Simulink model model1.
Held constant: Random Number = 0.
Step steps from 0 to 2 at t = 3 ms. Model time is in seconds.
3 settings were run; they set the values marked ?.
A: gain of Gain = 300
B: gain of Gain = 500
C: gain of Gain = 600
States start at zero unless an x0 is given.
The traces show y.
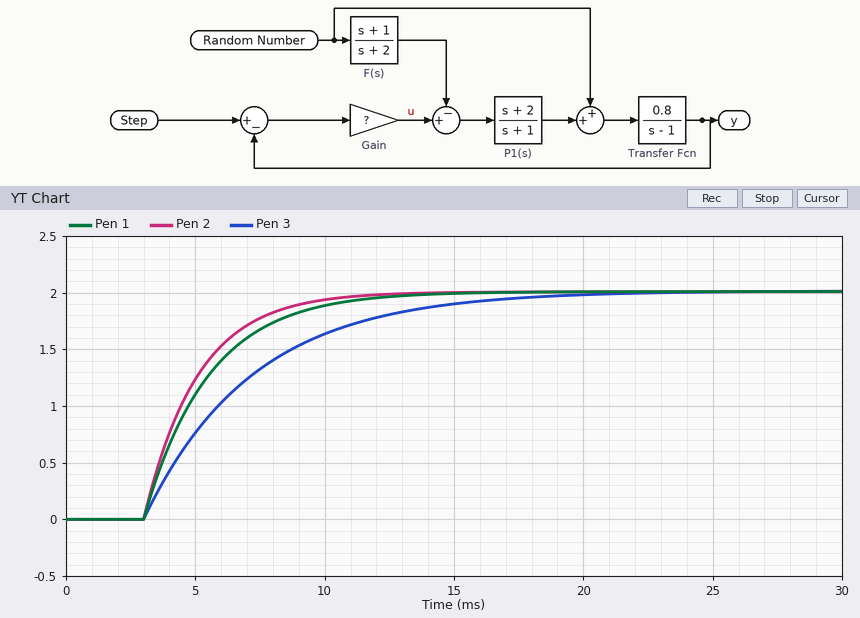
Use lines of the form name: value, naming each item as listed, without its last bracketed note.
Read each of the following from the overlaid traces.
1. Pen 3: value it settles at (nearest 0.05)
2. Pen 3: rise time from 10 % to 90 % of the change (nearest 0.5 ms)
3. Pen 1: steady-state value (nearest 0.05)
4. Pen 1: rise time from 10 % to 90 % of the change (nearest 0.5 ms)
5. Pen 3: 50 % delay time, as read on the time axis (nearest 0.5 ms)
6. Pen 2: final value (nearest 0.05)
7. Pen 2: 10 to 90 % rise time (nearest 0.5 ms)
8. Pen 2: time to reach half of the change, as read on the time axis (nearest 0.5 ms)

Pen 3: value it settles at: 2.00
Pen 3: rise time from 10 % to 90 % of the change: 9.0 ms
Pen 1: steady-state value: 2.00
Pen 1: rise time from 10 % to 90 % of the change: 5.5 ms
Pen 3: 50 % delay time, as read on the time axis: 6.0 ms
Pen 2: final value: 2.00
Pen 2: 10 to 90 % rise time: 4.5 ms
Pen 2: time to reach half of the change, as read on the time axis: 4.5 ms
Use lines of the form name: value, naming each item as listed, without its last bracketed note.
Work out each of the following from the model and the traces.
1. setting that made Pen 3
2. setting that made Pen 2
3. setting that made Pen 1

setting that made Pen 3: A
setting that made Pen 2: C
setting that made Pen 1: B
